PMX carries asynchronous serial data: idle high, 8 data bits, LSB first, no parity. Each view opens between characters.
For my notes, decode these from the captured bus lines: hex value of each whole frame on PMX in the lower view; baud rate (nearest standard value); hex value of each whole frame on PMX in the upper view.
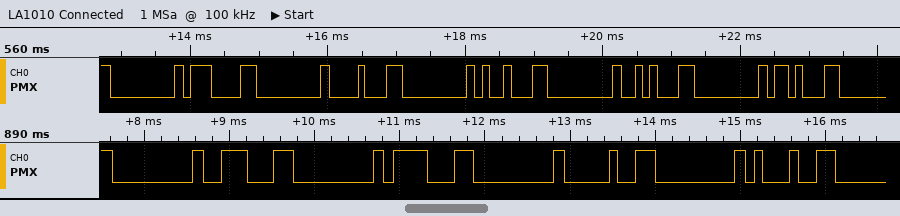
00, 8E, 00, 8F, 00, 90, 00, 91
9600 baud
00, 87, 00, 88, 00, 89, 00, 8A, 00, 8B
